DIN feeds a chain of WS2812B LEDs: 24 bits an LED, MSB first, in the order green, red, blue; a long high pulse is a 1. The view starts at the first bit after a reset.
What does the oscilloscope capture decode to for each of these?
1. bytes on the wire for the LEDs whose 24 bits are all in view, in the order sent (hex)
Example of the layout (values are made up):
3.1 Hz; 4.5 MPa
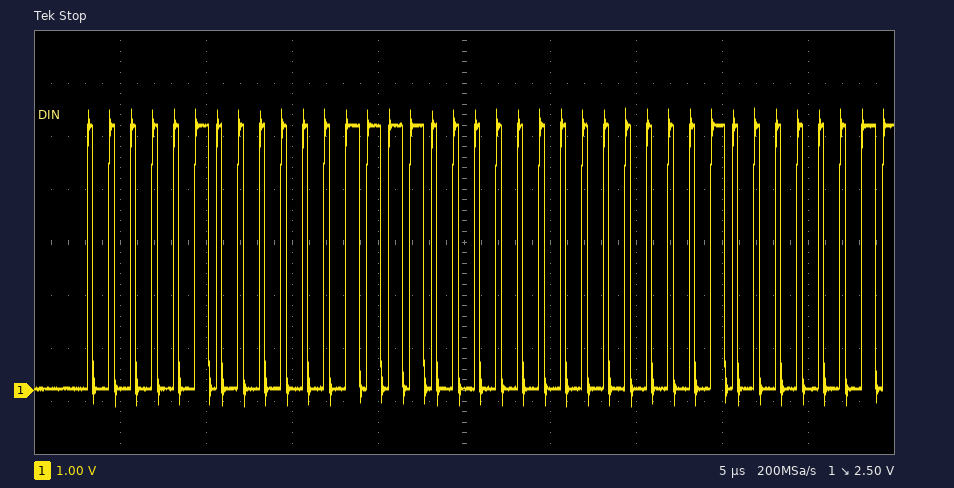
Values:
04 0F 00
